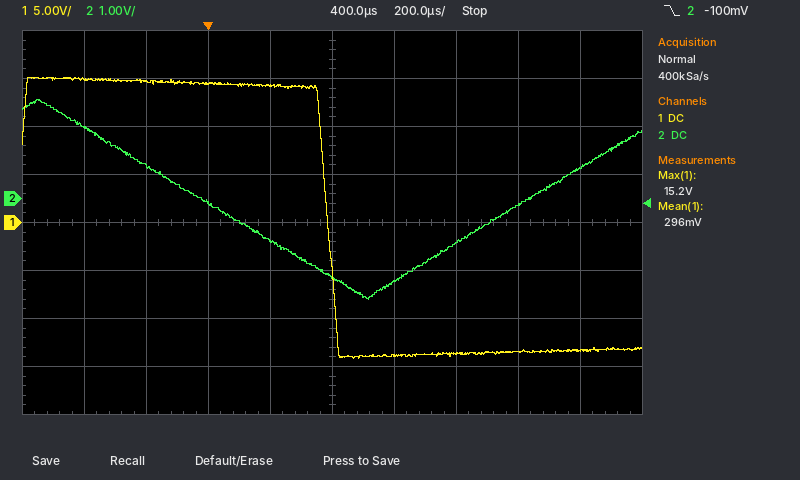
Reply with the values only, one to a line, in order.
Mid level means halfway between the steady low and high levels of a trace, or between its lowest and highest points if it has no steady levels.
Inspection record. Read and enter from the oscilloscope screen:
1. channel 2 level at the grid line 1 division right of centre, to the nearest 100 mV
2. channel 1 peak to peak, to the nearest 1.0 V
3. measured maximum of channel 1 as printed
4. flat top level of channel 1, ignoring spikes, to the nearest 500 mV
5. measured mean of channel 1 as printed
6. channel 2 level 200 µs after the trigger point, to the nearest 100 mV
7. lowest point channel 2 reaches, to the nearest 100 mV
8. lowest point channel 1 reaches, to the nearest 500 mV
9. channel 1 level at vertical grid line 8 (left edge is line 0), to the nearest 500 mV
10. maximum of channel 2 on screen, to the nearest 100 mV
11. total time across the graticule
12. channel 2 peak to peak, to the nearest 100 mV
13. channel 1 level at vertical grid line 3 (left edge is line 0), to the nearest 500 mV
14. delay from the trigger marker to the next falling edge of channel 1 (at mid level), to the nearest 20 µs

-1.7 V
29.0 V
15.2 V
14.5 V
296 mV
-900 mV
-2.1 V
-14.0 V
-13.5 V
2.1 V
2 ms
4.2 V
14.5 V
380 µs
